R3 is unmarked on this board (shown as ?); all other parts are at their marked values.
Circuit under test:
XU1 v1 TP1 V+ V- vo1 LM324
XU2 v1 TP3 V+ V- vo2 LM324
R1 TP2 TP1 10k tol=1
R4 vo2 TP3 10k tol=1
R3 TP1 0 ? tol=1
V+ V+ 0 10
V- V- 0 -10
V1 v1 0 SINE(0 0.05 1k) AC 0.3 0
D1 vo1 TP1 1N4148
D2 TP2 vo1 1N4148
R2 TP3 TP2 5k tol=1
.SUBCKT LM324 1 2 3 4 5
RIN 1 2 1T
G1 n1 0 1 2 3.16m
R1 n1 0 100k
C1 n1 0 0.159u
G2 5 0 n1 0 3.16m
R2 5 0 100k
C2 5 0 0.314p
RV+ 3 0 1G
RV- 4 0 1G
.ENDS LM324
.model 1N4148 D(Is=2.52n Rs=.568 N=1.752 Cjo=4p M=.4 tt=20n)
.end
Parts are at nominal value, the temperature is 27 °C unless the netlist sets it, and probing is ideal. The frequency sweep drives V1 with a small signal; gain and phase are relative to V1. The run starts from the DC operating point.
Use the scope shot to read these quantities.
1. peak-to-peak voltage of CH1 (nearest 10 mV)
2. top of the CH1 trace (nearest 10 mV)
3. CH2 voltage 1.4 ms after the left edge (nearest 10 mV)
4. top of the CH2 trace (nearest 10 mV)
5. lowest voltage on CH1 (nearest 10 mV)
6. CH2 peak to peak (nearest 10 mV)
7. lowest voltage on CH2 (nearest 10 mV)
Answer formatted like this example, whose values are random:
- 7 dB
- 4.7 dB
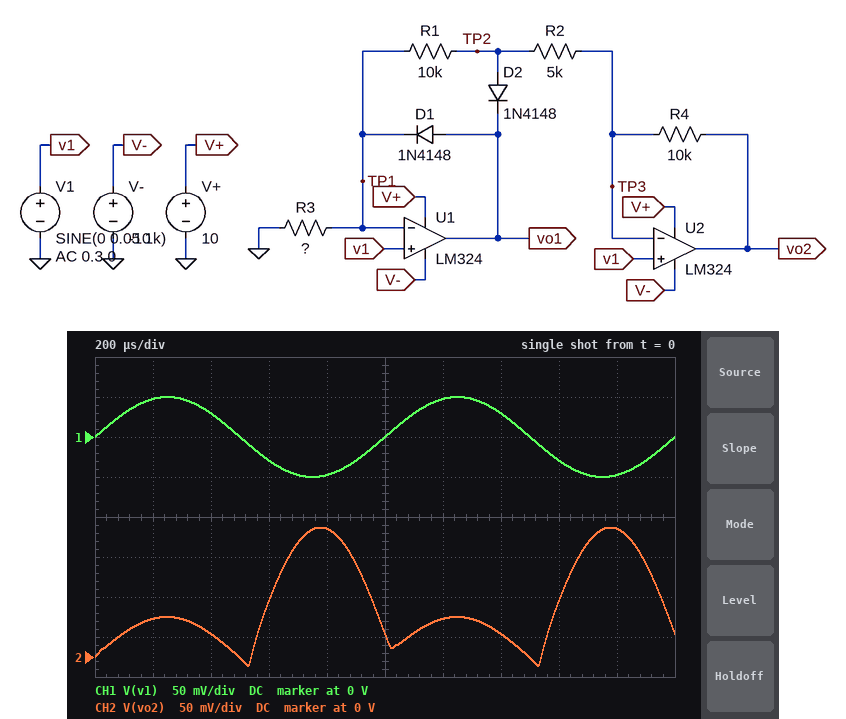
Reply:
- 100 mV
- 50 mV
- 30 mV
- 160 mV
- -50 mV
- 170 mV
- -10 mV
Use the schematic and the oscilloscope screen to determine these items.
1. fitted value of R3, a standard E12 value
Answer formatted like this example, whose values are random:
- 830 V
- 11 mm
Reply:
- 4.7 kΩ
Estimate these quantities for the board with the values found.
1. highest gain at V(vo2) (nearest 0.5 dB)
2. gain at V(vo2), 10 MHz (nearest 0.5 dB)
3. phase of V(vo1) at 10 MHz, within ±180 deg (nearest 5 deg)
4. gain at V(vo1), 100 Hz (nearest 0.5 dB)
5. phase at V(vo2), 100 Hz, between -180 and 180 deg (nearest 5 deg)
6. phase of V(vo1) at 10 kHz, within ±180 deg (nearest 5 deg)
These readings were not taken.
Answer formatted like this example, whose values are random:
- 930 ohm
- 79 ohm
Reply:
- 2.5 dB
- -33.5 dB
- -130 deg
- 68.0 dB
- 70 deg
- -90 deg
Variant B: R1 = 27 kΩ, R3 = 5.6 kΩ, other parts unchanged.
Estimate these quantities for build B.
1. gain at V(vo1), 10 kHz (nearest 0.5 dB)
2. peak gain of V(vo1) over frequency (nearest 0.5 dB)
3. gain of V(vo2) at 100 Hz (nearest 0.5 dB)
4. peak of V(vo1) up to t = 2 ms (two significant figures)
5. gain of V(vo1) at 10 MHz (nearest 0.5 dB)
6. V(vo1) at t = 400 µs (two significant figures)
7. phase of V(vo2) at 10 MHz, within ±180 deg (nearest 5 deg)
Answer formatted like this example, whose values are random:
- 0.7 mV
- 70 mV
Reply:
- 37.5 dB
- 68.5 dB
- -7.0 dB
- 420 mV
- -39.5 dB
- 380 mV
- -125 deg
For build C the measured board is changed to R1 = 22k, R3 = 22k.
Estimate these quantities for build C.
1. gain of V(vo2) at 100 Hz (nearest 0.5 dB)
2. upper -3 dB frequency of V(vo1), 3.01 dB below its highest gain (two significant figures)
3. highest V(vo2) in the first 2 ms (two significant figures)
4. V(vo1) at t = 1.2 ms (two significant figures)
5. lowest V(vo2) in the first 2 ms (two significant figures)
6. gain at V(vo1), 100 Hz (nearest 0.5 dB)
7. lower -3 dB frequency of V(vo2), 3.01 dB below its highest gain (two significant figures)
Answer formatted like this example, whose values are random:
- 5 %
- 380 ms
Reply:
- -3.0 dB
- 590 Hz
- 50 mV
- 350 mV
- -9.7 mV
- 56.5 dB
- 270 Hz
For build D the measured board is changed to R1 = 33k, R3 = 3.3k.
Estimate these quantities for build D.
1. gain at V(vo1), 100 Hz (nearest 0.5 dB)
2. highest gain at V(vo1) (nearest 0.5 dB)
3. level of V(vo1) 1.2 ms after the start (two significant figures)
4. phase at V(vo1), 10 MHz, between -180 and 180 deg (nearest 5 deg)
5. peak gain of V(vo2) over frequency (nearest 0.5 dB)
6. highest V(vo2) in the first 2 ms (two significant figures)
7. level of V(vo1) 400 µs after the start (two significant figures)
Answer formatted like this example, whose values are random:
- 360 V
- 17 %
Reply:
- 72.0 dB
- 73.0 dB
- 440 mV
- -140 deg
- 1.5 dB
- 910 mV
- 400 mV
